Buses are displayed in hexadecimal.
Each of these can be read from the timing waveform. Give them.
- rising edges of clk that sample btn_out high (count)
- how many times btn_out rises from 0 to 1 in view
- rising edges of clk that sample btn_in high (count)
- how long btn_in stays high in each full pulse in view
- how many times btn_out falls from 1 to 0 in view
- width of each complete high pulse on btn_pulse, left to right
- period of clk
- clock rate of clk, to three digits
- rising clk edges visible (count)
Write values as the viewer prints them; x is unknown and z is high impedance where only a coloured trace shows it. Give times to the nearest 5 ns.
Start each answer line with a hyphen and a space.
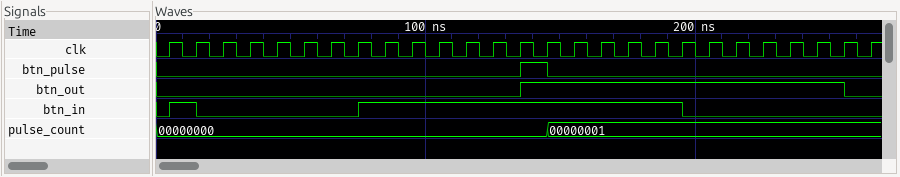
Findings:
- 12
- 1
- 13
- 10 ns, 120 ns
- 1
- 10 ns
- 10 ns
- 100 MHz
- 27
